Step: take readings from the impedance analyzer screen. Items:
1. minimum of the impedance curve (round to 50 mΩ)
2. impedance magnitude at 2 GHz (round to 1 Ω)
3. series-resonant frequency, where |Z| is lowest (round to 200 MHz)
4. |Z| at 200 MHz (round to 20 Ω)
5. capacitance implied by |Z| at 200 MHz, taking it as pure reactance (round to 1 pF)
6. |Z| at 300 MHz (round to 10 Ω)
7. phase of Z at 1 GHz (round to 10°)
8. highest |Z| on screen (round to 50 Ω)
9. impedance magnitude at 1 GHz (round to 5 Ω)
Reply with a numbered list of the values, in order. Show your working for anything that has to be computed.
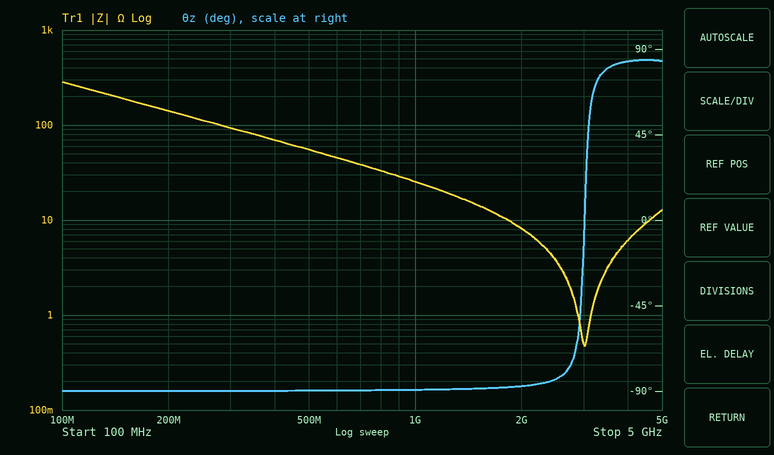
1. 450 mΩ
2. 8 Ω
3. 3.0 GHz
4. 140 Ω
5. C = 1/(2π × 200 MHz × 140 Ω) ≈ 6 pF
6. 90 Ω
7. -90°
8. 300 Ω
9. 25 Ω
